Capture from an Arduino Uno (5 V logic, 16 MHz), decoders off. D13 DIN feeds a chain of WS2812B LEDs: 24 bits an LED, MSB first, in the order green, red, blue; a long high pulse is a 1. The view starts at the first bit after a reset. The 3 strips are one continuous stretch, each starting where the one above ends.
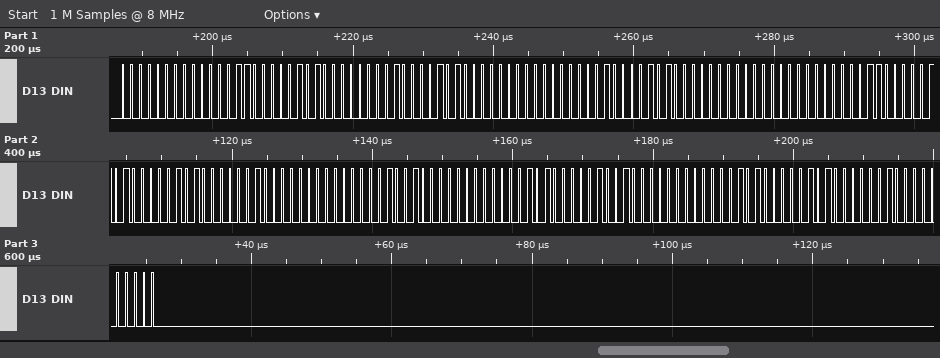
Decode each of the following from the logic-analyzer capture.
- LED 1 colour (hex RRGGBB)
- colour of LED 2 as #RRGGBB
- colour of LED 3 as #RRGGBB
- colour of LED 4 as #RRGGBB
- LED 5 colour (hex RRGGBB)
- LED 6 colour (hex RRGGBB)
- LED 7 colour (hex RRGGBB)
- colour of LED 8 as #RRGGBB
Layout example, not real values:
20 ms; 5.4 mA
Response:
#06000A; #0A0100; #0A0100; #06000A; #040A00; #00090A; #00090A; #040A00
